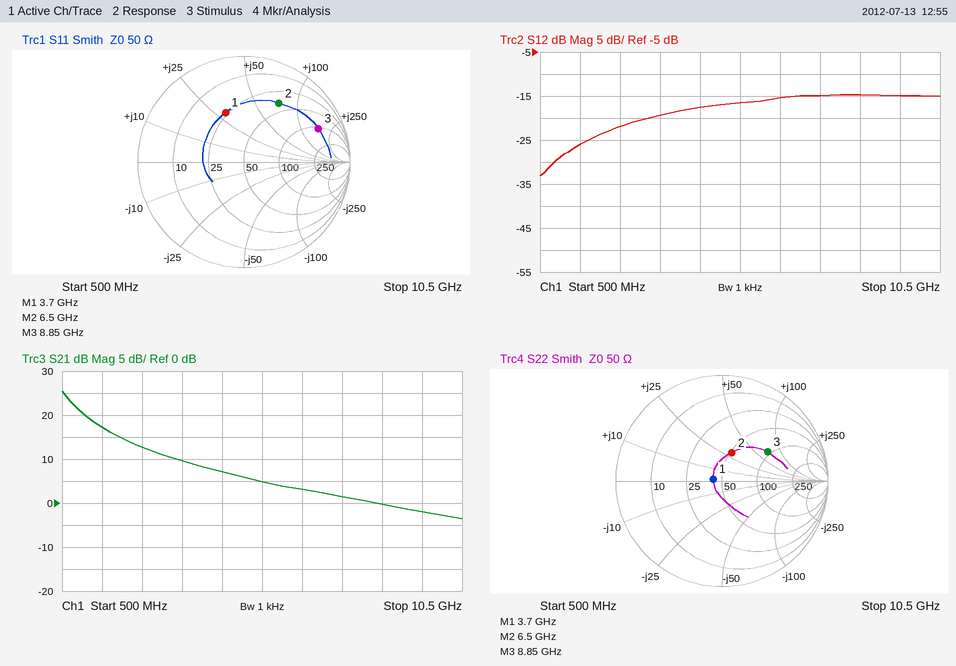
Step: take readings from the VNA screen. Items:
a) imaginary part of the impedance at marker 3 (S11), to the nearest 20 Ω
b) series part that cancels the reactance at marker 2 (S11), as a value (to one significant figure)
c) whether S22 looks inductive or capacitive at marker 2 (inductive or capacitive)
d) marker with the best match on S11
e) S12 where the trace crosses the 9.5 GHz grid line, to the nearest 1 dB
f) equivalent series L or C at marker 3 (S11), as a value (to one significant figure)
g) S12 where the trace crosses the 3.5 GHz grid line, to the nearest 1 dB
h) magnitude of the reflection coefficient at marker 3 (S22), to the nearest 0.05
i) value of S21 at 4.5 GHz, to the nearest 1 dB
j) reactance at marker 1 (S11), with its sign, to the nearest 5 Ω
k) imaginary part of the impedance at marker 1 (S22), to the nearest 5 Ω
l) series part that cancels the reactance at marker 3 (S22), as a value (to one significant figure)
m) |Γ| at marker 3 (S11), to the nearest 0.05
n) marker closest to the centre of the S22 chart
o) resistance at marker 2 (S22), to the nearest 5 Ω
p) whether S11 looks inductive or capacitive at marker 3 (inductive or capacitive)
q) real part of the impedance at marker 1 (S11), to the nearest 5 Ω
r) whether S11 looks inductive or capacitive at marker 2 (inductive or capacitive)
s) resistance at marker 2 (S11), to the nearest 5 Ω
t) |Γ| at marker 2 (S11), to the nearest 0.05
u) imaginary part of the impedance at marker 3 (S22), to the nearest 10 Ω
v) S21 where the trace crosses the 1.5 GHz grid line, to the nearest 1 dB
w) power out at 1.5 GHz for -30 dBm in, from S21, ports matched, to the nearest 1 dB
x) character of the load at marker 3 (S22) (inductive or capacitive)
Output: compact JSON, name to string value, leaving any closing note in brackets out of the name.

{"imaginary part of the impedance at marker 3 (S11), to the nearest 20 Ω": "+160 Ω", "series part that cancels the reactance at marker 2 (S11), as a value": "300 fF", "whether S22 looks inductive or capacitive at marker 2": "inductive", "marker with the best match on S11": "marker 1", "S12 where the trace crosses the 9.5 GHz grid line, to the nearest 1 dB": "-15 dB", "equivalent series L or C at marker 3 (S11), as a value": "3 nH", "S12 where the trace crosses the 3.5 GHz grid line, to the nearest 1 dB": "-19 dB", "magnitude of the reflection coefficient at marker 3 (S22), to the nearest 0.05": "0.50", "value of S21 at 4.5 GHz, to the nearest 1 dB": "7 dB", "reactance at marker 1 (S11), with its sign, to the nearest 5 Ω": "+30 Ω", "imaginary part of the impedance at marker 1 (S22), to the nearest 5 Ω": "0 Ω", "series part that cancels the reactance at marker 3 (S22), as a value": "300 fF", "|Γ| at marker 3 (S11), to the nearest 0.05": "0.75", "marker closest to the centre of the S22 chart": "marker 1", "resistance at marker 2 (S22), to the nearest 5 Ω": "50 Ω", "whether S11 looks inductive or capacitive at marker 3": "inductive", "real part of the impedance at marker 1 (S11), to the nearest 5 Ω": "25 Ω", "whether S11 looks inductive or capacitive at marker 2": "inductive", "resistance at marker 2 (S11), to the nearest 5 Ω": "40 Ω", "|Γ| at marker 2 (S11), to the nearest 0.05": "0.65", "imaginary part of the impedance at marker 3 (S22), to the nearest 10 Ω": "+70 Ω", "S21 where the trace crosses the 1.5 GHz grid line, to the nearest 1 dB": "17 dB", "power out at 1.5 GHz for -30 dBm in, from S21, ports matched, to the nearest 1 dB": "-13 dBm", "character of the load at marker 3 (S22)": "inductive"}
